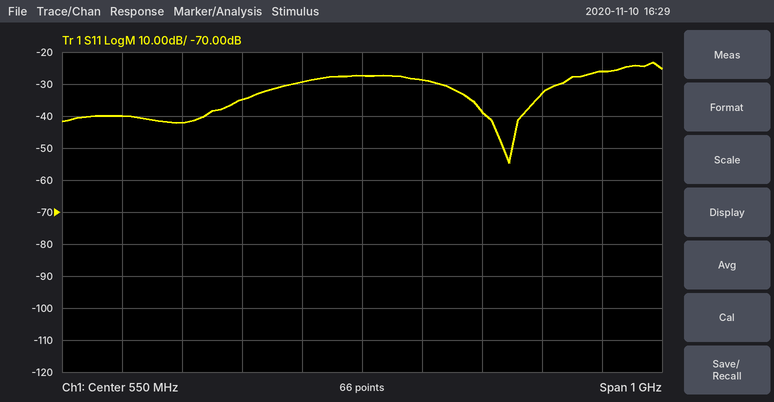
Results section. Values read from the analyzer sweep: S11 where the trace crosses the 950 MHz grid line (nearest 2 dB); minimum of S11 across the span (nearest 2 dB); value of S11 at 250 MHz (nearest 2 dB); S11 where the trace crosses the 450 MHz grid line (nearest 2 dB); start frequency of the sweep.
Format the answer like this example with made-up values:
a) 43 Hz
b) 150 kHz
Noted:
a) -26 dB
b) -54 dB
c) -42 dB
d) -30 dB
e) 50 MHz
